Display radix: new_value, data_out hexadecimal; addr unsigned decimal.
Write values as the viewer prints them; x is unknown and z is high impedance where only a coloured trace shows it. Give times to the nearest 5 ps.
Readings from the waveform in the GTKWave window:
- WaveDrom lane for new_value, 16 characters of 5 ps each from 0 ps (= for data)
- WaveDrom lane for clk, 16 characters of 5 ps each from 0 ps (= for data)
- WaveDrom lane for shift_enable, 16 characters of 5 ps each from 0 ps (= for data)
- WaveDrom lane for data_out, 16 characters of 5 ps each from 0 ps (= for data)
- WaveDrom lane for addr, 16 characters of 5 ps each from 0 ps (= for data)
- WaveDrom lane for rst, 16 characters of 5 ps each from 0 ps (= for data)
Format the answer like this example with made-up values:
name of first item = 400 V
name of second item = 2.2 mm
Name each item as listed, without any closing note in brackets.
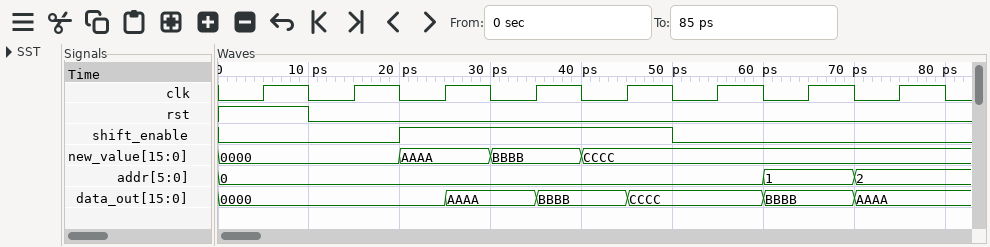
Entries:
WaveDrom lane for new_value, 16 characters of 5 ps each from 0 ps = {name: 'new_value', wave: '=...=.=.=.......', data: '0000 AAAA BBBB CCCC'}
WaveDrom lane for clk, 16 characters of 5 ps each from 0 ps = {name: 'clk', wave: '0101010101010101'}
WaveDrom lane for shift_enable, 16 characters of 5 ps each from 0 ps = {name: 'shift_enable', wave: '0...1.....0.....'}
WaveDrom lane for data_out, 16 characters of 5 ps each from 0 ps = {name: 'data_out', wave: '=....=.=.=..=.=.', data: '0000 AAAA BBBB CCCC BBBB AAAA'}
WaveDrom lane for addr, 16 characters of 5 ps each from 0 ps = {name: 'addr', wave: '=...........=.=.', data: '0 1 2'}
WaveDrom lane for rst, 16 characters of 5 ps each from 0 ps = {name: 'rst', wave: '1.0.............'}
